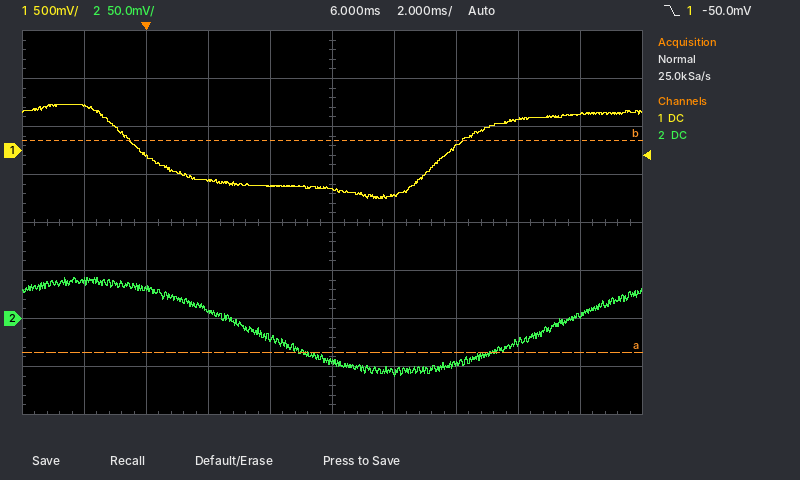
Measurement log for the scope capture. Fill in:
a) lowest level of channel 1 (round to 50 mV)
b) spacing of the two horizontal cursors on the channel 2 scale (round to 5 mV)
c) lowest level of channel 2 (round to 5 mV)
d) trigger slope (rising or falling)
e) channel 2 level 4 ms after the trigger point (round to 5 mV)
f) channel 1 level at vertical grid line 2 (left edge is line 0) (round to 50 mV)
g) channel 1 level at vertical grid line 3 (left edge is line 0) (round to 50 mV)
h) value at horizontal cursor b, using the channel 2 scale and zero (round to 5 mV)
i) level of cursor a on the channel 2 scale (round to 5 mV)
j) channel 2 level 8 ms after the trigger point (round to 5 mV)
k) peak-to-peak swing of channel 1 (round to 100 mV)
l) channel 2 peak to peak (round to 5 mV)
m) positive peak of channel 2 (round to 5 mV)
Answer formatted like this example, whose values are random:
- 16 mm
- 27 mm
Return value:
- -500 mV
- 220 mV
- -60 mV
- falling
- -20 mV
- -50 mV
- -300 mV
- 185 mV
- -35 mV
- -55 mV
- 1.00 V
- 105 mV
- 45 mV
